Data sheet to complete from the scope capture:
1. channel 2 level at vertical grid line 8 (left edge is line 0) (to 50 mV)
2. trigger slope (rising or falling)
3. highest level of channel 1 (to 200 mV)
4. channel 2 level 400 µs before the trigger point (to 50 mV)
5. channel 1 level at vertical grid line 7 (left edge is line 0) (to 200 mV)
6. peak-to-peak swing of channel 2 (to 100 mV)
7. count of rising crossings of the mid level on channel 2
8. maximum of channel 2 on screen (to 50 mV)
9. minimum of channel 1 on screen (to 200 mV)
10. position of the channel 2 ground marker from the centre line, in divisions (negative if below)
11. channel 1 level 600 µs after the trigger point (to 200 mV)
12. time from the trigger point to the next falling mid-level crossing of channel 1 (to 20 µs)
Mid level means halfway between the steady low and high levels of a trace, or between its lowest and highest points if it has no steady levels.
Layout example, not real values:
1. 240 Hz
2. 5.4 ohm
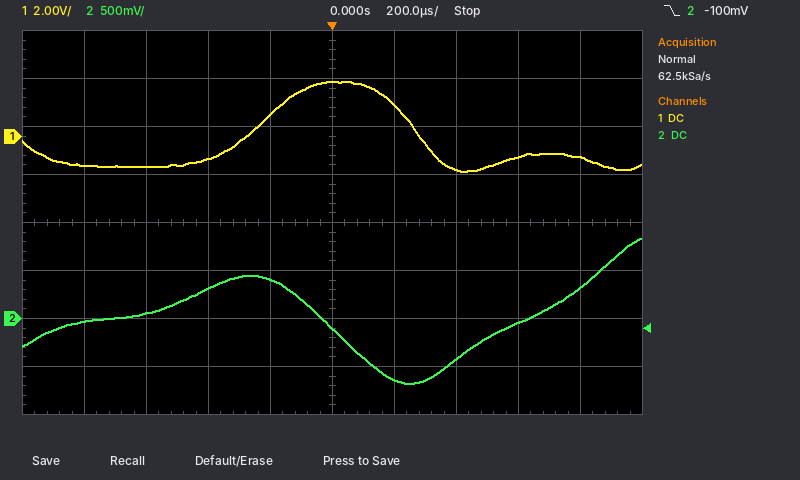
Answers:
1. -50 mV
2. falling
3. 2.2 V
4. 300 mV
5. -1.4 V
6. 1.50 V
7. 2
8. 850 mV
9. -1.4 V
10. -2.0 div
11. -800 mV
12. 260 µs
